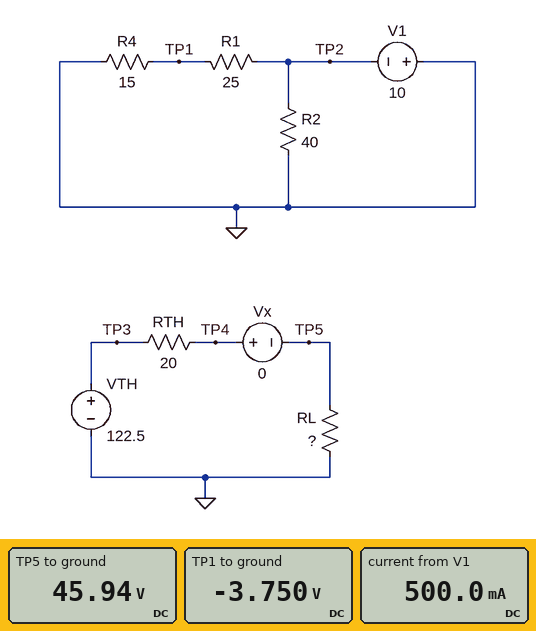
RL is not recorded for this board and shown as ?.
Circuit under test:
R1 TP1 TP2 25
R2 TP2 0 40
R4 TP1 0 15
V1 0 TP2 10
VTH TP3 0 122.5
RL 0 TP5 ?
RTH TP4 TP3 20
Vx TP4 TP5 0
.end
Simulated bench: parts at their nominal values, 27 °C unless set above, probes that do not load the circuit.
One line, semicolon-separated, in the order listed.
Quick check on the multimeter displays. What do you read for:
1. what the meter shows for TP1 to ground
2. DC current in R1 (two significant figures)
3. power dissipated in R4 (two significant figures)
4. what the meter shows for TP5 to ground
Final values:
-3.750 V; 250 mA; 940 mW; 45.94 V
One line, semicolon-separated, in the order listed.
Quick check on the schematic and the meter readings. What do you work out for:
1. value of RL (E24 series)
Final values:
12 Ω
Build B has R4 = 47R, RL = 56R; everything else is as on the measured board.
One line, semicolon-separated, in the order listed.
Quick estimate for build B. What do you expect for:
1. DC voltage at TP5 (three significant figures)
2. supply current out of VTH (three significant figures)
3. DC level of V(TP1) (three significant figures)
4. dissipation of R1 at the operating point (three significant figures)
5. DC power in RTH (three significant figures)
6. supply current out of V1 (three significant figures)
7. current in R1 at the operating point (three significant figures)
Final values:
90.3 V; 1.61 A; -6.53 V; 482 mW; 52.0 W; 389 mA; 139 mA
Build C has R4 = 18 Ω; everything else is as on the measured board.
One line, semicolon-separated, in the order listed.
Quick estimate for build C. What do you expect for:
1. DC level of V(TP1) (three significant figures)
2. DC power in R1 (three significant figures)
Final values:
-4.19 V; 1.35 W
